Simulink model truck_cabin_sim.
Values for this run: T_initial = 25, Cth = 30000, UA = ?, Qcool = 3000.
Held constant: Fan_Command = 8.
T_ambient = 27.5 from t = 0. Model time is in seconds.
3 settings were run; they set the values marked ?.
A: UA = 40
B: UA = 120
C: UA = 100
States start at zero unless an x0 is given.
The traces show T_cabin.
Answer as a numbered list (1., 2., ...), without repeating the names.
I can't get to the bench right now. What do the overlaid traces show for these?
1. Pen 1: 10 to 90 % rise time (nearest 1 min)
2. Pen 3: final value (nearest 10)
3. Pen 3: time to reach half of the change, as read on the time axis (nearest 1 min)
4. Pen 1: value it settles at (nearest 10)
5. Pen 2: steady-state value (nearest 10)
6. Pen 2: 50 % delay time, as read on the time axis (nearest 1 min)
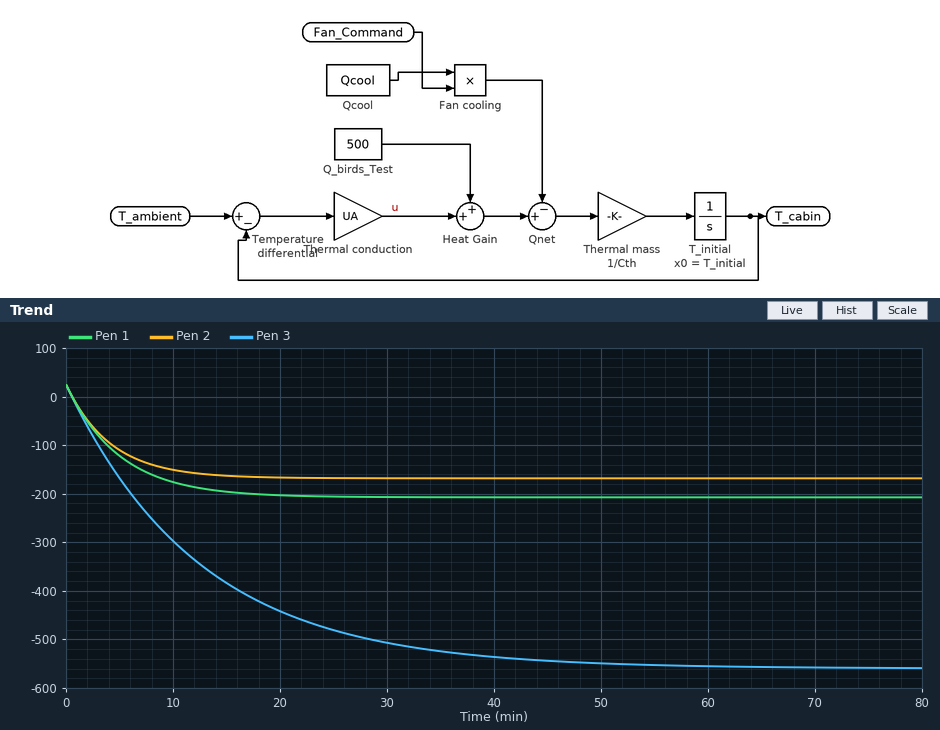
1. 11 min
2. -560
3. 9 min
4. -210
5. -170
6. 3 min
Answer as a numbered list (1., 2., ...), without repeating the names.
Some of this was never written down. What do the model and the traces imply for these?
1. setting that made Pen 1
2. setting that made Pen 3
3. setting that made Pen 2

1. C
2. A
3. B
